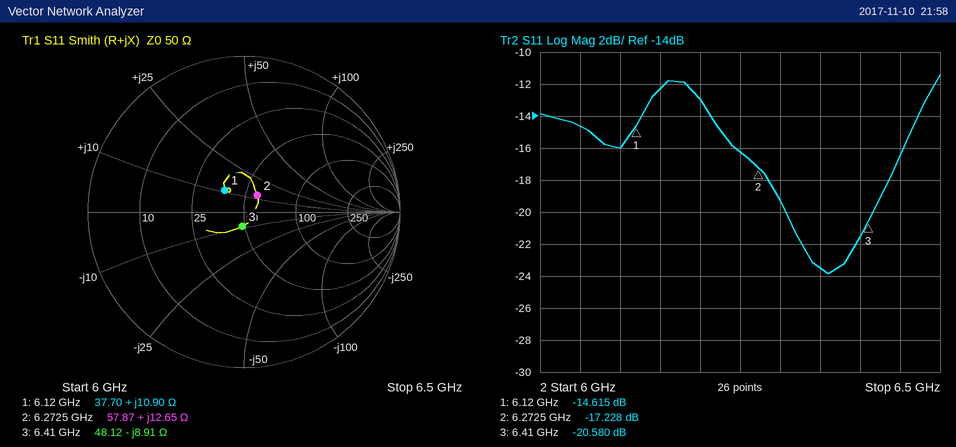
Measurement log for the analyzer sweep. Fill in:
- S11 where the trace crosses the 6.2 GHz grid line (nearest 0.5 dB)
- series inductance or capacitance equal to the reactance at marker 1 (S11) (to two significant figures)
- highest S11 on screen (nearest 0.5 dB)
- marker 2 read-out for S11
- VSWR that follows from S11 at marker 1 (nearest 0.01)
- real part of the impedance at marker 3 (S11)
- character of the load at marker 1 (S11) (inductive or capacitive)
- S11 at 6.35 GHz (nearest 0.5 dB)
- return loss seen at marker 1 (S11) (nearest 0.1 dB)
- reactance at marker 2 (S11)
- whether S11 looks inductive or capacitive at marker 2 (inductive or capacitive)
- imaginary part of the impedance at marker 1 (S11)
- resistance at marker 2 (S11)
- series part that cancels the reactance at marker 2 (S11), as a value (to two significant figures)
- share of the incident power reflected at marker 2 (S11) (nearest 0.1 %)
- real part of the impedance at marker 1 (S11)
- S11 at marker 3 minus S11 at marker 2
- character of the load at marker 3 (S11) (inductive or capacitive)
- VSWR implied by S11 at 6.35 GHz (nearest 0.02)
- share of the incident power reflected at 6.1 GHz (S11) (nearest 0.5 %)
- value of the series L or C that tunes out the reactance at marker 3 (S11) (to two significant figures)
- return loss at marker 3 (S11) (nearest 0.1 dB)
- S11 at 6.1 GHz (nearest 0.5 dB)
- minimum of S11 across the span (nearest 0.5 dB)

-13.0 dB
280 pH
-11.5 dB
-17.228 dB
1.46
48.12 Ω
inductive
-23.5 dB
14.6 dB
+12.65 Ω
inductive
+10.90 Ω
57.87 Ω
2.0 pF
1.9 %
37.70 Ω
-3.352 dB
capacitive
1.14
2.5 %
220 pH
20.7 dB
-16.0 dB
-24.0 dB
